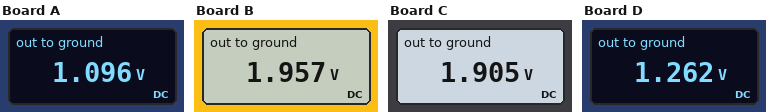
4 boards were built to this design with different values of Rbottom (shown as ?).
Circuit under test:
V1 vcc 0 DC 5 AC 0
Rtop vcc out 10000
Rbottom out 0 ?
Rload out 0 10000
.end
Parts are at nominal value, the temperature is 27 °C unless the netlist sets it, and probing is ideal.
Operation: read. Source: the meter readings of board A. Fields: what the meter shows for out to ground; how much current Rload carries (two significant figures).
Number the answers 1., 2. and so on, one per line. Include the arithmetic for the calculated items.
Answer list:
1. 1.096 V
2. (1.096 V) / 10 kΩ = 110 µA
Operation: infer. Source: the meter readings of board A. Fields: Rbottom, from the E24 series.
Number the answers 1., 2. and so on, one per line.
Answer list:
1. 3.9 kΩ
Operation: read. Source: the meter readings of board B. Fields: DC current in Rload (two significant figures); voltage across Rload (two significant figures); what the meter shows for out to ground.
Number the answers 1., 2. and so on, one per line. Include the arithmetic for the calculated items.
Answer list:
1. (1.957 V) / 10 kΩ = 200 µA
2. 1.957 V = 2.0 V
3. 1.957 V
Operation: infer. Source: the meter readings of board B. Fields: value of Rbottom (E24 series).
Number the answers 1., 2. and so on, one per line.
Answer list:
1. 18 kΩ
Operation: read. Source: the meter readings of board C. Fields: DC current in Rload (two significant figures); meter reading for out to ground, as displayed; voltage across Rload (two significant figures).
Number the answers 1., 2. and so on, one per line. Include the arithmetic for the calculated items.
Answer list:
1. (1.905 V) / 10 kΩ = 190 µA
2. 1.905 V
3. 1.905 V = 1.9 V
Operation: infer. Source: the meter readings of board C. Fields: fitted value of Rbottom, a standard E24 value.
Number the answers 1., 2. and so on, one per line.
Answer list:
1. 16 kΩ
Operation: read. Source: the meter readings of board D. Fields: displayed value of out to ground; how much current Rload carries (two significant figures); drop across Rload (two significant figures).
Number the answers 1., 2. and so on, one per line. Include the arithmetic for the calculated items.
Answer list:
1. 1.262 V
2. (1.262 V) / 10 kΩ = 130 µA
3. 1.262 V = 1.3 V
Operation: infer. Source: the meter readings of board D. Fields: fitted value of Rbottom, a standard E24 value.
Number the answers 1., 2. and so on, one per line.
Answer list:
1. 5.1 kΩ
